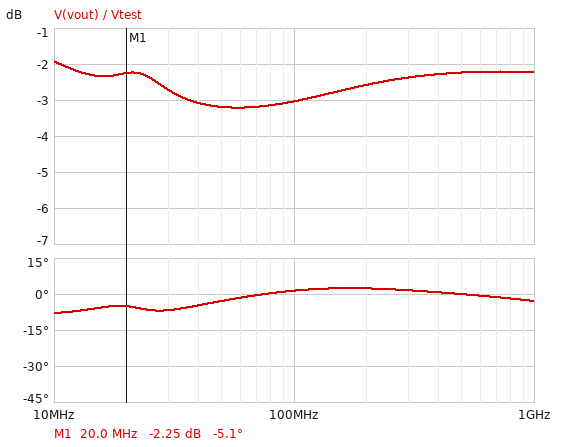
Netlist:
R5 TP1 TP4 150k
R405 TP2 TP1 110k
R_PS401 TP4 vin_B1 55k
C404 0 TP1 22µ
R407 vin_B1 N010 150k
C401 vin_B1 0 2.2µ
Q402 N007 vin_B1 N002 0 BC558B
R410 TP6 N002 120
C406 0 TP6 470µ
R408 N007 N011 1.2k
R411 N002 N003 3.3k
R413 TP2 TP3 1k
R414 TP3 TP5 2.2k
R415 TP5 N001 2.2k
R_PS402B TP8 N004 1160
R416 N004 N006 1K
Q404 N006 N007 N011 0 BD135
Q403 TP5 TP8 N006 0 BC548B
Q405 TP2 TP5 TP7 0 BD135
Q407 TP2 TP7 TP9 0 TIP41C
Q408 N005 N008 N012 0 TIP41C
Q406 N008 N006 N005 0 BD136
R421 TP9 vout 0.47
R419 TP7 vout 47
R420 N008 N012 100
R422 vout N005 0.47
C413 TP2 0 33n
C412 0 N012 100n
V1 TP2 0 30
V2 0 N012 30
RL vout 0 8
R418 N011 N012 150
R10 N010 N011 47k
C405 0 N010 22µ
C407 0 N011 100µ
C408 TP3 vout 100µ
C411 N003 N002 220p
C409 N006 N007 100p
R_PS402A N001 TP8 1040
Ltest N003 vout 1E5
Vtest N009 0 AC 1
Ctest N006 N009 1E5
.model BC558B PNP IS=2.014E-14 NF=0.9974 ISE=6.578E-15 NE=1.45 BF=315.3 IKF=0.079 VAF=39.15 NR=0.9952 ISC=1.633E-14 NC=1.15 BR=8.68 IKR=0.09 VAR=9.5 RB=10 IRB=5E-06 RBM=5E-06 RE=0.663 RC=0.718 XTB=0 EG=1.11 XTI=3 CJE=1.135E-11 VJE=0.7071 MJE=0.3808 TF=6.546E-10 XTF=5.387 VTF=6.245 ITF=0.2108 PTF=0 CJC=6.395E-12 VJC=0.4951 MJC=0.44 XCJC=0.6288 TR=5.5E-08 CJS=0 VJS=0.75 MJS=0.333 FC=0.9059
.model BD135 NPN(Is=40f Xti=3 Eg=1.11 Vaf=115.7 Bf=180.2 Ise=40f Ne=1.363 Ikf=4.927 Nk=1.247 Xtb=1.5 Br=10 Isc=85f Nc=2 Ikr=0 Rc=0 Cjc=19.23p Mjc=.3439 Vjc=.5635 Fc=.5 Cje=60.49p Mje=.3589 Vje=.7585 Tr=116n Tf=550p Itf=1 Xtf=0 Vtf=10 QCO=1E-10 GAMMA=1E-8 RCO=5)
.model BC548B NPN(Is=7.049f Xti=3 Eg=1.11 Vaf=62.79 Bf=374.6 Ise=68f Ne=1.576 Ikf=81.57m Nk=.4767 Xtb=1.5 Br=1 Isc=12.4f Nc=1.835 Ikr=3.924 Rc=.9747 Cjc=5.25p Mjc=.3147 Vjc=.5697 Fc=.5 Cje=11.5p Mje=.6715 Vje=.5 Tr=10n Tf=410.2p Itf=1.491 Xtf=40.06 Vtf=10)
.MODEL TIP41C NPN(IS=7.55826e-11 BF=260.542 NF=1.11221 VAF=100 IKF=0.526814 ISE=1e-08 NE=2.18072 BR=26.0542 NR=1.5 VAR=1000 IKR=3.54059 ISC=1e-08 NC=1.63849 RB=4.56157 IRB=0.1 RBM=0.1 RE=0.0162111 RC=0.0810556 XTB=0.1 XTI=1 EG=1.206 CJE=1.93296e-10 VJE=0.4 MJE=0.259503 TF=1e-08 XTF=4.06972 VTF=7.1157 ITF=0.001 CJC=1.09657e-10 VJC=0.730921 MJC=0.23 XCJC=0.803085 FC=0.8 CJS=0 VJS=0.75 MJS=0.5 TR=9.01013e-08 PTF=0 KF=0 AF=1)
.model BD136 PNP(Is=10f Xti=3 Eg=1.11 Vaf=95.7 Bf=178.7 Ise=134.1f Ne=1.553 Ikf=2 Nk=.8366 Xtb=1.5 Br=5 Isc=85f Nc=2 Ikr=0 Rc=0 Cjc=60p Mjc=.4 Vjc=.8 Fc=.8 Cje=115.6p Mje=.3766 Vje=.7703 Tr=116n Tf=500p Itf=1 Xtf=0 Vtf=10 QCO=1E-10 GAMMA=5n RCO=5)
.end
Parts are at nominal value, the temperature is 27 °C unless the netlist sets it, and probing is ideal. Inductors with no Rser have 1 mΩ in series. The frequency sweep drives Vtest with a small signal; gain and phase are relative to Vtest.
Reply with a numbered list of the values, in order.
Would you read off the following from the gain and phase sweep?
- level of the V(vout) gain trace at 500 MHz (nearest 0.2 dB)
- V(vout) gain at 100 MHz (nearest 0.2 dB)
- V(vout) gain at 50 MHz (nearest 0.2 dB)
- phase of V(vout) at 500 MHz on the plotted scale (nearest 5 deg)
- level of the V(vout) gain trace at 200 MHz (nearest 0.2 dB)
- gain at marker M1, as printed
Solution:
1. -2.2 dB
2. -3.0 dB
3. -3.2 dB
4. 0 deg
5. -2.6 dB
6. -2.25 dB
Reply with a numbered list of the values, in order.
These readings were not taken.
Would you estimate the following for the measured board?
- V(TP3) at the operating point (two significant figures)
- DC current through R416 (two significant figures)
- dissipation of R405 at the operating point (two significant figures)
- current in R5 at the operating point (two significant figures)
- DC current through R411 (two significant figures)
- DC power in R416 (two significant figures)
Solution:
1. 20 V
2. 340 µA
3. 1.4 mW
4. 110 µA
5. 620 µA
6. 110 µW
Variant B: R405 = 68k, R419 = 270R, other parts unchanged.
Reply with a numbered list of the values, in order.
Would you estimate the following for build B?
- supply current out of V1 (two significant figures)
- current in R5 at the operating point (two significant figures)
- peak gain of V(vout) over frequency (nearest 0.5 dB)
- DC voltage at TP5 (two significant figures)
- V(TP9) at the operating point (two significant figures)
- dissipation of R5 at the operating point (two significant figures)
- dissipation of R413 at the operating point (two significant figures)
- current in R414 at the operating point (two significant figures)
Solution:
1. 15 mA
2. 120 µA
3. -0.5 dB
4. -51 mV
5. -1.2 V
6. 2.3 mW
7. 88 mW
8. 9.4 mA
